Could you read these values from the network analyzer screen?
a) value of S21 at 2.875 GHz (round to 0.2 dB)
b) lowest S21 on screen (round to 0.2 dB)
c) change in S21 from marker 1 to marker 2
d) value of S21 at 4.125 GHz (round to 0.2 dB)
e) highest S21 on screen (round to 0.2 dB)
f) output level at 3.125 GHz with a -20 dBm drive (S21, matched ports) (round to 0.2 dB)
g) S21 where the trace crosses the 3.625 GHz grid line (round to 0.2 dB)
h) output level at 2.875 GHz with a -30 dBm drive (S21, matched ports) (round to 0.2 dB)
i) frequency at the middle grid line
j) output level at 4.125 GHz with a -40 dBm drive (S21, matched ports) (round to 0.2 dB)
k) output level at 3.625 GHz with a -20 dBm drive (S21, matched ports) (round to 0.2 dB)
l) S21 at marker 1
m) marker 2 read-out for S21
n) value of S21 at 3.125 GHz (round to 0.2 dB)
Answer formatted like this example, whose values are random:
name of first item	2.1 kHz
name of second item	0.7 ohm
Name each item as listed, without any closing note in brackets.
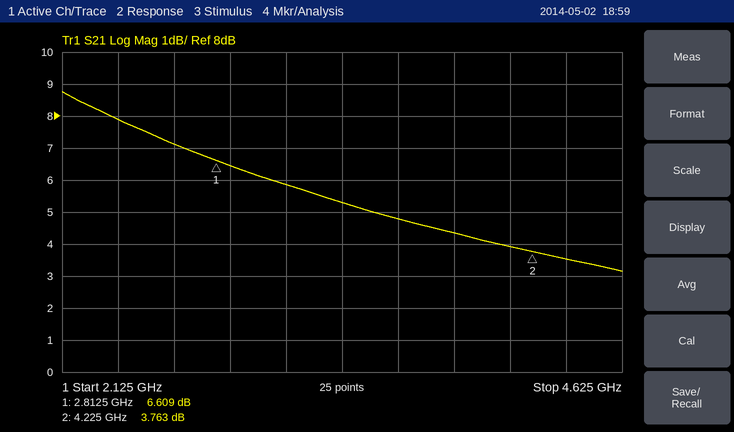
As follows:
value of S21 at 2.875 GHz	6.4 dB
lowest S21 on screen	3.2 dB
change in S21 from marker 1 to marker 2	-2.846 dB
value of S21 at 4.125 GHz	4.0 dB
highest S21 on screen	8.8 dB
output level at 3.125 GHz with a -20 dBm drive (S21, matched ports)	-14.2 dBm
S21 where the trace crosses the 3.625 GHz grid line	4.8 dB
output level at 2.875 GHz with a -30 dBm drive (S21, matched ports)	-23.6 dBm
frequency at the middle grid line	3.375 GHz
output level at 4.125 GHz with a -40 dBm drive (S21, matched ports)	-36.0 dBm
output level at 3.625 GHz with a -20 dBm drive (S21, matched ports)	-15.2 dBm
S21 at marker 1	6.609 dB
marker 2 read-out for S21	3.763 dB
value of S21 at 3.125 GHz	5.8 dB
